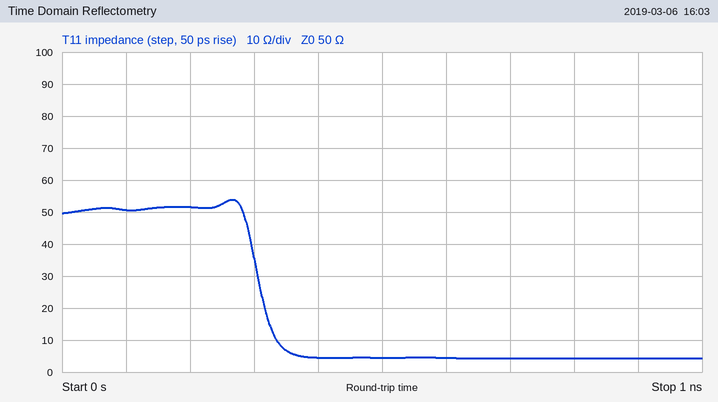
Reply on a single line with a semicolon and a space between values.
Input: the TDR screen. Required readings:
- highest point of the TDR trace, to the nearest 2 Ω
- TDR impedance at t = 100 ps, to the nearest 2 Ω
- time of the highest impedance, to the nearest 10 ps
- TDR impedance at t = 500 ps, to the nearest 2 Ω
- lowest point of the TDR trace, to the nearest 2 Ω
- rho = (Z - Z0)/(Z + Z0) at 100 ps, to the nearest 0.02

54 Ω; 50 Ω; 270 ps; 4 Ω; 4 Ω; 0.00
